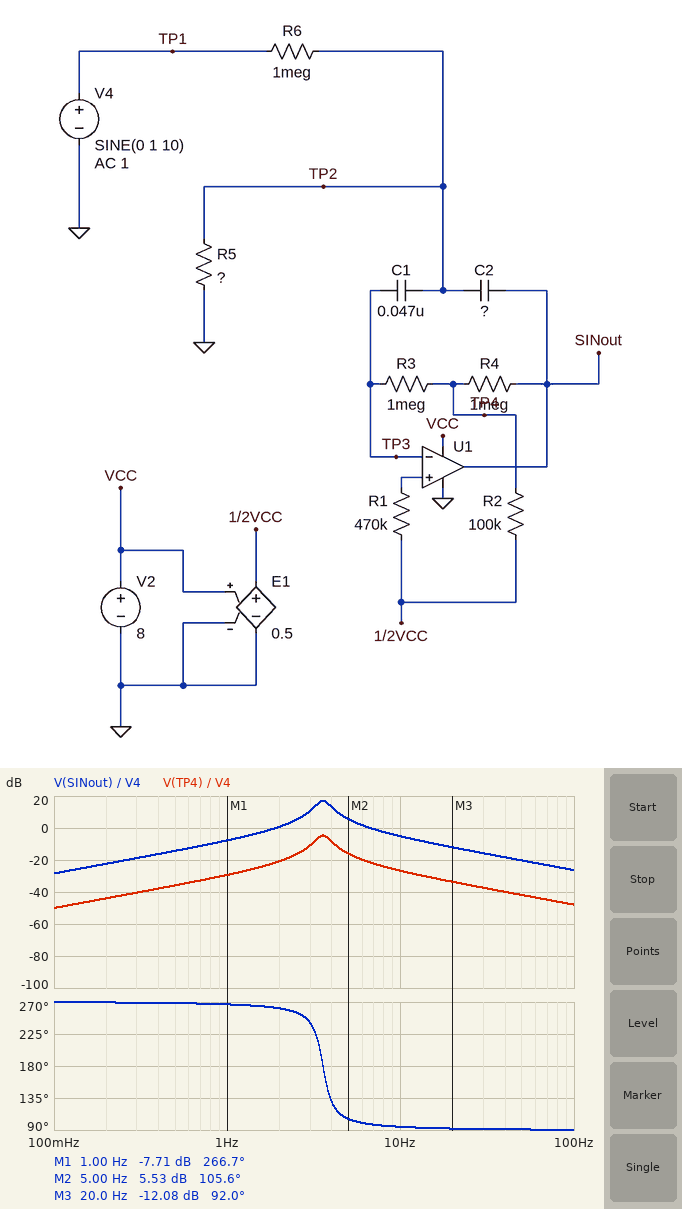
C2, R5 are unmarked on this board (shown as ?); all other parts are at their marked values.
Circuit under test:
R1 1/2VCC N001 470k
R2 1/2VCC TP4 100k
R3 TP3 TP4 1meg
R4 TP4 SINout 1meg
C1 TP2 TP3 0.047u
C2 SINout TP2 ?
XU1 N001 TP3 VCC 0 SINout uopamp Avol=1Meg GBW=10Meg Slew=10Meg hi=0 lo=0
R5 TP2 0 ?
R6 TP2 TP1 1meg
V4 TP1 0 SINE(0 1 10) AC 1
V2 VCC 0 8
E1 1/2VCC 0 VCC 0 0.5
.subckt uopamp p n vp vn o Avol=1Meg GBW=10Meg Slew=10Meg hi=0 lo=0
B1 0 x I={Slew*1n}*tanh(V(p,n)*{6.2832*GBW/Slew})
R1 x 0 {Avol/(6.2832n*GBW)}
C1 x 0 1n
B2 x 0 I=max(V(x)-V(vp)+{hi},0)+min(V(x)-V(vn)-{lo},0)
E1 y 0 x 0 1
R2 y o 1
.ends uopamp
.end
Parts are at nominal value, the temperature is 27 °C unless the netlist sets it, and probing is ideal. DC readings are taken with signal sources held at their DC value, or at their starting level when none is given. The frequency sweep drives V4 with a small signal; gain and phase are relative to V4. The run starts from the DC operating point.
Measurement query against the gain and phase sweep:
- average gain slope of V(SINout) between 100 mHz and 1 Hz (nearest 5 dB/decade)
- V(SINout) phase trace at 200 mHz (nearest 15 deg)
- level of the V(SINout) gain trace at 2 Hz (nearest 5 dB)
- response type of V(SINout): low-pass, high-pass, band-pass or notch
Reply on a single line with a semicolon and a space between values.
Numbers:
20 dB/decade; 270 deg; 0 dB; band-pass
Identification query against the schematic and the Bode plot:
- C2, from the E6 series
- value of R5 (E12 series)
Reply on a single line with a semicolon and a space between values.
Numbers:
33 nF; 120 kΩ
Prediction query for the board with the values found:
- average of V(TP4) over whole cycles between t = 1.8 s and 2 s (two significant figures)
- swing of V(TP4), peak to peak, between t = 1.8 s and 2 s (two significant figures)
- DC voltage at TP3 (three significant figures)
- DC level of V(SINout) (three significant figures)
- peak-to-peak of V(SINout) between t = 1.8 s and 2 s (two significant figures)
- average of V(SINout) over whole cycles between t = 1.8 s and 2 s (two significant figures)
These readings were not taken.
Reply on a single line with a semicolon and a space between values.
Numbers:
4.0 V; 93 mV; 4.00 V; 4.00 V; 1.1 V; 4.0 V
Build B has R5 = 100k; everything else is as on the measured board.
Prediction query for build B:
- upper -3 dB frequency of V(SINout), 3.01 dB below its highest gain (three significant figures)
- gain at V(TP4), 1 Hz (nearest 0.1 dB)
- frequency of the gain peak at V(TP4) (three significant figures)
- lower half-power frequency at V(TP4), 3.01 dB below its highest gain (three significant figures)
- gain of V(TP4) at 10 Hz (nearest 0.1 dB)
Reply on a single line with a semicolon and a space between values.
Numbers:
4.23 Hz; -30.8 dB; 3.87 Hz; 3.54 Hz; -26.5 dB
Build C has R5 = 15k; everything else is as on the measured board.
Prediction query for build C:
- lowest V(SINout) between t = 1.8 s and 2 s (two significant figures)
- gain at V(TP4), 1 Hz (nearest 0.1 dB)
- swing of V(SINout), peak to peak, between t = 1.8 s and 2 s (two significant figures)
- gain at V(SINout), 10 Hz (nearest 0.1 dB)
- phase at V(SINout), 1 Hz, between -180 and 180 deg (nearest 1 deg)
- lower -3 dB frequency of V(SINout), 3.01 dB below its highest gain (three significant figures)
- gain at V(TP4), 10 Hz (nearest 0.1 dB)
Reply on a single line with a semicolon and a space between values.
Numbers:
-1.5 mV; -47.1 dB; 8.0 V; 13.3 dB; -90 deg; 9.26 Hz; -8.3 dB
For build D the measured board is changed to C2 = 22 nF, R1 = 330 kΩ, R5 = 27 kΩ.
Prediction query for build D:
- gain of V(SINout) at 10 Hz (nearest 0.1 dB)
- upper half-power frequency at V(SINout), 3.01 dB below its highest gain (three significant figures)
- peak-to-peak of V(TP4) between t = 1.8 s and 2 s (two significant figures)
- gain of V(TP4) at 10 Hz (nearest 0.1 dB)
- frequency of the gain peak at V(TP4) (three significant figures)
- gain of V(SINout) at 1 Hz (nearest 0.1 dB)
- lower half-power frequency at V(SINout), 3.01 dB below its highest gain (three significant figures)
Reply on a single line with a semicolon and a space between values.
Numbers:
9.6 dB; 9.27 Hz; 500 mV; -12.0 dB; 8.81 Hz; -20.5 dB; 8.38 Hz
